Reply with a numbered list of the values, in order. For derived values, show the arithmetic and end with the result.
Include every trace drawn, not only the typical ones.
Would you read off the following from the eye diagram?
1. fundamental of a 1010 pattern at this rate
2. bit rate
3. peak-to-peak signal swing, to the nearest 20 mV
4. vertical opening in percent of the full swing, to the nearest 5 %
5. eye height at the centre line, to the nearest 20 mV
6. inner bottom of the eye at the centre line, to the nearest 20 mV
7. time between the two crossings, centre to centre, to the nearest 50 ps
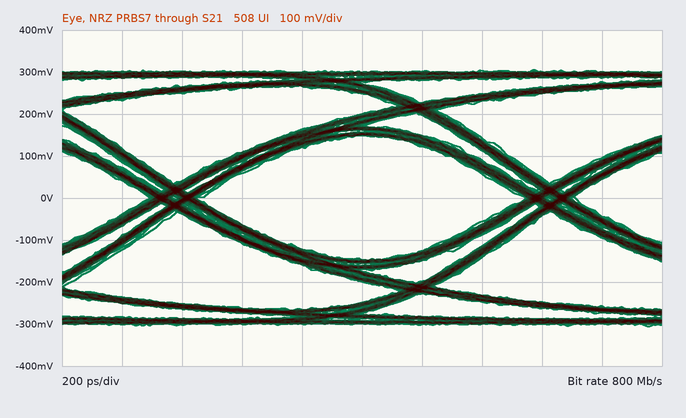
1. 400 MHz
2. 800 Mb/s
3. 620 mV
4. 300 mV / 620 mV ≈ 48.4 %, so 50 % to the nearest 5 %
5. 300 mV
6. -140 mV
7. 1.25 ns
